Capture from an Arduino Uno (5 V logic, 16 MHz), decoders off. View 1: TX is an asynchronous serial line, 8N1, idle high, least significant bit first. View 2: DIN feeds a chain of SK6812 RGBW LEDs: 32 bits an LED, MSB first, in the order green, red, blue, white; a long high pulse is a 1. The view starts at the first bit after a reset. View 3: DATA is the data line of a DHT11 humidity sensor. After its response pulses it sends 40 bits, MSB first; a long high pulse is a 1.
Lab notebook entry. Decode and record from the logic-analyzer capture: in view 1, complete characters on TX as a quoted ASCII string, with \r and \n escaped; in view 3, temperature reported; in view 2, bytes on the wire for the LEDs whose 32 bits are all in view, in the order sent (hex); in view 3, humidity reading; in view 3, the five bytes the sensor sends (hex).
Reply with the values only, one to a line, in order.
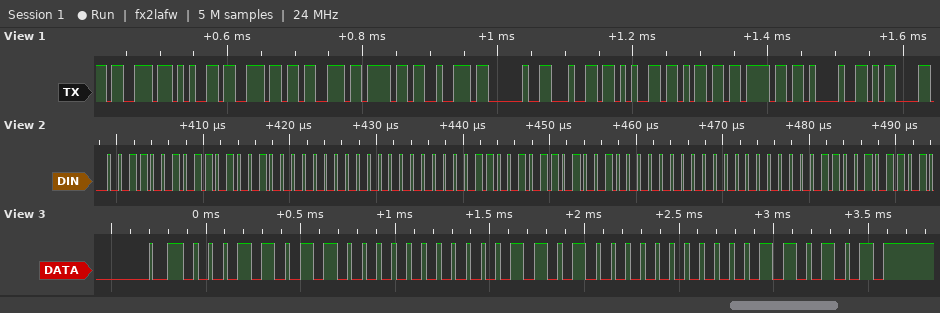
"sensor demo!\r"
26.0 °C
32 D2 00 00 32 D2 00 00
27 %
1B 00 1A 00 35
